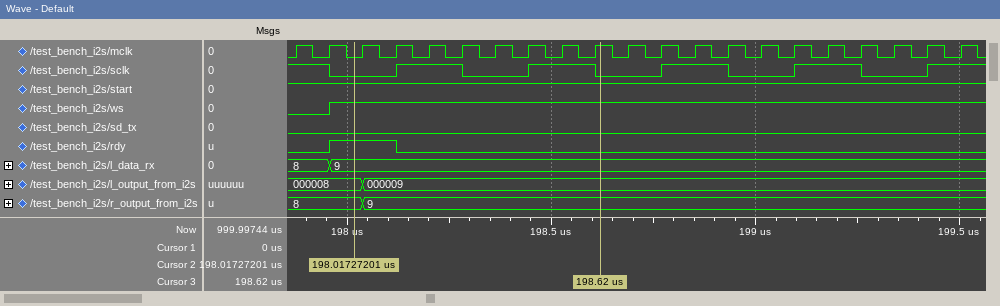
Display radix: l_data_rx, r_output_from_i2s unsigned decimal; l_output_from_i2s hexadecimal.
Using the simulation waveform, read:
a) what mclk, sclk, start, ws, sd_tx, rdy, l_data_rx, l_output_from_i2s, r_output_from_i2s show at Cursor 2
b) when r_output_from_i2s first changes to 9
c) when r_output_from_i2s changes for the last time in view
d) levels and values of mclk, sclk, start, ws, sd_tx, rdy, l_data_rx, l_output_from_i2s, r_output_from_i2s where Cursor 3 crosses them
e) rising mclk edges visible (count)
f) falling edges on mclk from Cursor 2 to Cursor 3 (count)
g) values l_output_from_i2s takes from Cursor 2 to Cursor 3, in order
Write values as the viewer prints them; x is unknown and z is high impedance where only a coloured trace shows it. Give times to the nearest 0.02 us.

mclk=0, sclk=0, start=1, ws=1, sd_tx=0, rdy=1, l_data_rx=9, l_output_from_i2s=000008, r_output_from_i2s=8
198.04 us
198.04 us
mclk=1, sclk=0, start=1, ws=1, sd_tx=0, rdy=0, l_data_rx=9, l_output_from_i2s=000009, r_output_from_i2s=9
21
7
000008, 000009
